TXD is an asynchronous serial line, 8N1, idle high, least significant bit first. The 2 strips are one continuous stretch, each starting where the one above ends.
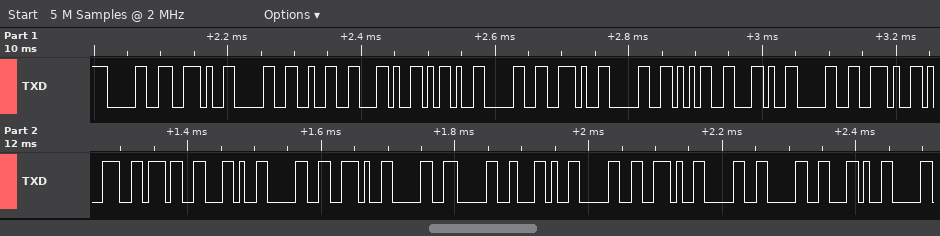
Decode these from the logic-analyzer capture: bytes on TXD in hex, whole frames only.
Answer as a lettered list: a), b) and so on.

a) 0x30 0x2E 0x30 0x32 0x2C 0x2D 0x30 0x2E 0x30 0x35 0x2C 0x30 0x2E 0x39 0x37 0x2C 0x30 0x2E 0x30 0x30 0x2C 0x30 0x2E 0x30 0x30 0x2C
